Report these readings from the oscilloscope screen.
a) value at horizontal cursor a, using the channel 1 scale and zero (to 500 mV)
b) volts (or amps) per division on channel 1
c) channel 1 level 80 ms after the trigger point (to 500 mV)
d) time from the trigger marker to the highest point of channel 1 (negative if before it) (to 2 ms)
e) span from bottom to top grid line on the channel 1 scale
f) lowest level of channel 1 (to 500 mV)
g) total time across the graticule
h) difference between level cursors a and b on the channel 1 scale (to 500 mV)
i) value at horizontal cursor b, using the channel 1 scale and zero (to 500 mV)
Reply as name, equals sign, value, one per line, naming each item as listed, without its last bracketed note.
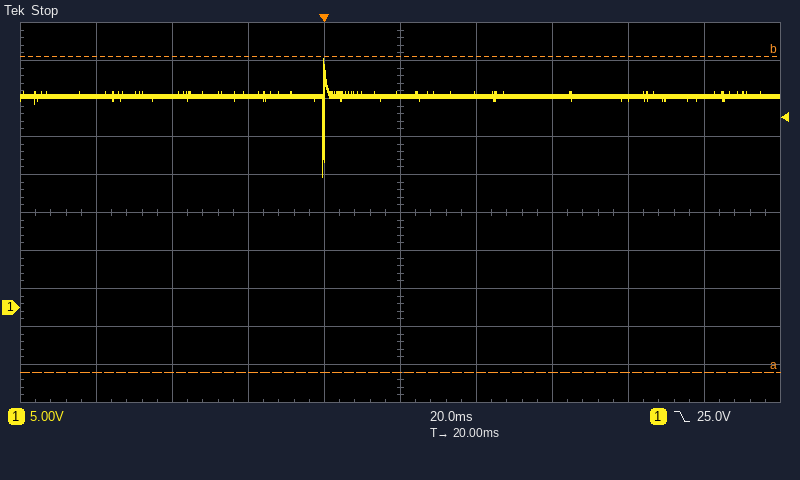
value at horizontal cursor a, using the channel 1 scale and zero = -8.5 V
volts (or amps) per division on channel 1 = 5 V
channel 1 level 80 ms after the trigger point = 27.5 V
time from the trigger marker to the highest point of channel 1 (negative if before it) = 0 ms
span from bottom to top grid line on the channel 1 scale = 50 V
lowest level of channel 1 = 17.0 V
total time across the graticule = 200 ms
difference between level cursors a and b on the channel 1 scale = 41.5 V
value at horizontal cursor b, using the channel 1 scale and zero = 33.0 V
